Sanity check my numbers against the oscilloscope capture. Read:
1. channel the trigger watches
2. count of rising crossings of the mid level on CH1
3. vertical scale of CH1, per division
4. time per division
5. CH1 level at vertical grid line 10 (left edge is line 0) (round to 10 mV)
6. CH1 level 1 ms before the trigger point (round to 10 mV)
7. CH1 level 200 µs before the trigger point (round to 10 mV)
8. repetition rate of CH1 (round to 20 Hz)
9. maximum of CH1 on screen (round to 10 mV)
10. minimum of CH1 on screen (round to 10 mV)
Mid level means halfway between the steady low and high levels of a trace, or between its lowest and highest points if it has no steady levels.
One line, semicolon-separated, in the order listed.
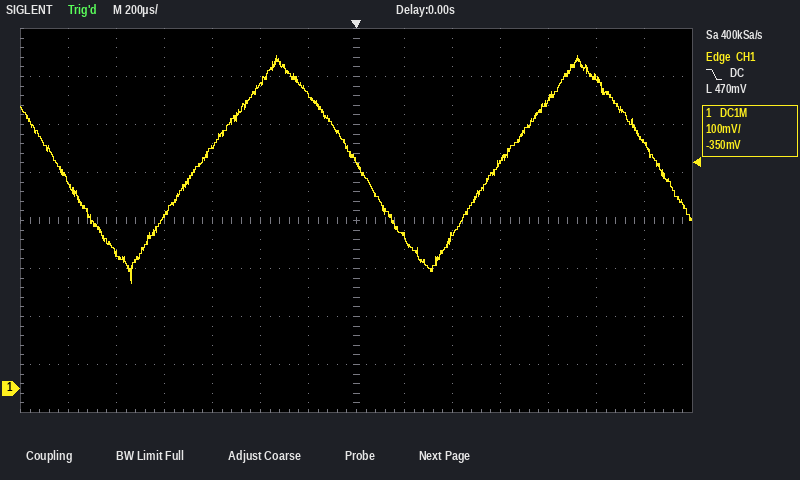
CH1; 2; 100 mV; 200 µs; 470 mV; 280 mV; 610 mV; 800 Hz; 690 mV; 220 mV
